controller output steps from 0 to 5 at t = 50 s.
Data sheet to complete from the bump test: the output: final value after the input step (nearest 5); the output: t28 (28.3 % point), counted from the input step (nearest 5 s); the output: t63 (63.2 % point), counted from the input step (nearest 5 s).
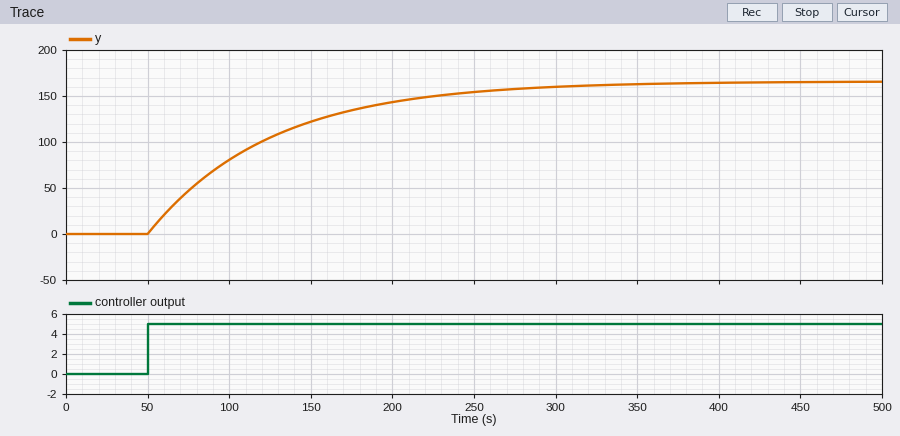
165
25 s
75 s
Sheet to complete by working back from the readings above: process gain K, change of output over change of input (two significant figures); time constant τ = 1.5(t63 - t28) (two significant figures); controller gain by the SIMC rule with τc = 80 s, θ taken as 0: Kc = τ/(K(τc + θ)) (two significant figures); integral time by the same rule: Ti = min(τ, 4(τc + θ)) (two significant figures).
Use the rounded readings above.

33
75 s
0.028
75 s
